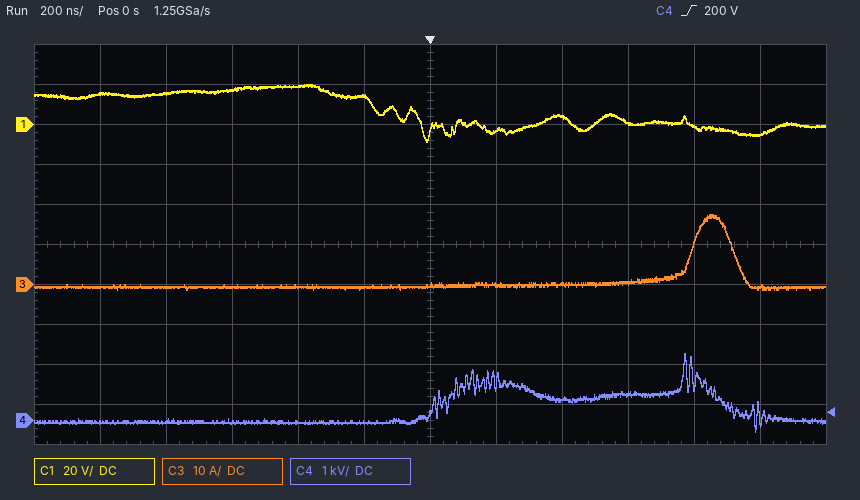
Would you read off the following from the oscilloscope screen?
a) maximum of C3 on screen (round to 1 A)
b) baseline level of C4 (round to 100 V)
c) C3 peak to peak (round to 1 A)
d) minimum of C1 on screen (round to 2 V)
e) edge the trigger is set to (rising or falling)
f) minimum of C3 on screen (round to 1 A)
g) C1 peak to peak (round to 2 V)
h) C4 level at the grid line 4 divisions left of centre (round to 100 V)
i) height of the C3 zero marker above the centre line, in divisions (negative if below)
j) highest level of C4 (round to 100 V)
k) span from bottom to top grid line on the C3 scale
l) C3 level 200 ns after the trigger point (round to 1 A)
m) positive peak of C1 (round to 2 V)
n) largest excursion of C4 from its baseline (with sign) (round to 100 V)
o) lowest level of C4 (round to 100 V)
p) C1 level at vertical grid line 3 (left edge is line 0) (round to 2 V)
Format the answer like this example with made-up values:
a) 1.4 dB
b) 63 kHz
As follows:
a) 18 A
b) 0.0 kV
c) 19 A
d) -8 V
e) rising
f) -1 A
g) 28 V
h) 0.0 kV
i) -1.0 div
j) 1.7 kV
k) 100 A
l) 0 A
m) 20 V
n) +1.7 kV
o) -300 V
p) 18 V
